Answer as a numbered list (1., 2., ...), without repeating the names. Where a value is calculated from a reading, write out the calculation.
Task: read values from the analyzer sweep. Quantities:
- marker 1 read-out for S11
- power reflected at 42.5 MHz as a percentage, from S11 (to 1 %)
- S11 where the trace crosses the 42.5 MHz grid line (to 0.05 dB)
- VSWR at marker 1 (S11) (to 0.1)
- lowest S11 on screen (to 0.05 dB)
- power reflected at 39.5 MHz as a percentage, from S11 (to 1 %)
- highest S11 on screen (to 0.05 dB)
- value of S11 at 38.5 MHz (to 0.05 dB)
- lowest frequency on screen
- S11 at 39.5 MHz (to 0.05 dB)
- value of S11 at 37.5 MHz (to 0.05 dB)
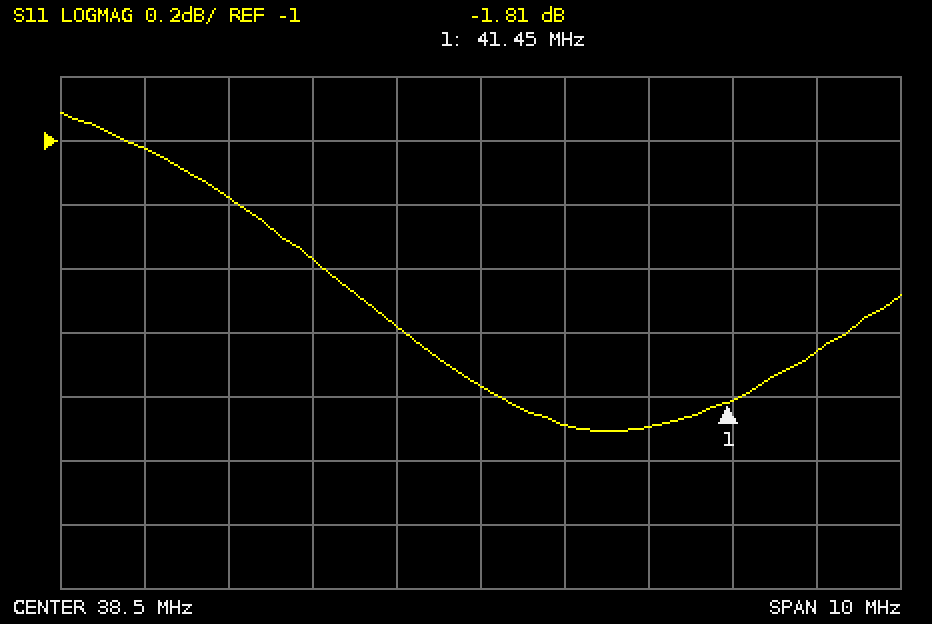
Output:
1. -1.81 dB
2. 10^(-1.65/10) ≈ 68 %
3. -1.65 dB
4. (1 + 0.8119)/(1 − 0.8119) ≈ 9.6
5. -1.90 dB
6. 10^(-1.9/10) ≈ 65 %
7. -0.90 dB
8. -1.75 dB
9. 33.5 MHz
10. -1.90 dB
11. -1.60 dB
